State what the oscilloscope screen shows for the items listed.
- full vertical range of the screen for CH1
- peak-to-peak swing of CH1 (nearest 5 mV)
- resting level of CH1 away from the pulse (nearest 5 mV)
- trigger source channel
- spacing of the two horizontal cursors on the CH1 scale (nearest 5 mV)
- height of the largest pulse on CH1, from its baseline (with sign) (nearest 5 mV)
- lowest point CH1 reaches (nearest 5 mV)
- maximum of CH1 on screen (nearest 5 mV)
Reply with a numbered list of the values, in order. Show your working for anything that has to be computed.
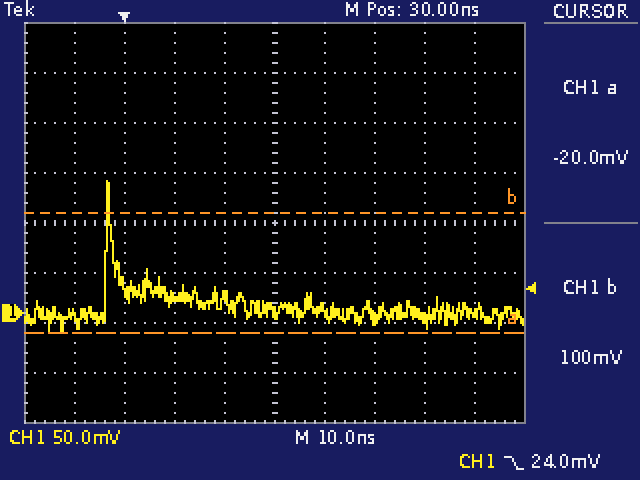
1. 400 mV
2. 130 mV − (-20 mV) = 150 mV
3. 0 mV
4. CH1
5. 120 mV
6. 130 mV − (0 mV) = +130 mV
7. -20 mV
8. 130 mV
